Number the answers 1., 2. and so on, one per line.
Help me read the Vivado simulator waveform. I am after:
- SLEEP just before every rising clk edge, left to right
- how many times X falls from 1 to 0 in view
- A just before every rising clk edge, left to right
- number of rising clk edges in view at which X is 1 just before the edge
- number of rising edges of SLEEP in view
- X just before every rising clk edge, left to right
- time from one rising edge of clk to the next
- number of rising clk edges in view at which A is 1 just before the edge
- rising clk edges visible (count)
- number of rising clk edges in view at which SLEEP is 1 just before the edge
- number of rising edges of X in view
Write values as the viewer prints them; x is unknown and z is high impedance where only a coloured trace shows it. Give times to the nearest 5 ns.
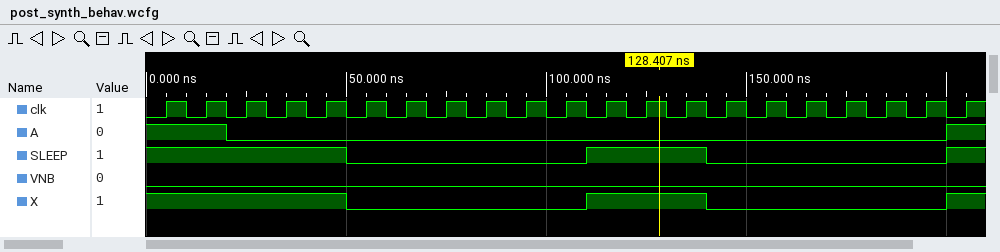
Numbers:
1. 1 1 1 1 1 0 0 0 0 0 0 1 1 1 0 0 0 0 0 0 1
2. 2
3. 1 1 0 0 0 0 0 0 0 0 0 0 0 0 0 0 0 0 0 0 1
4. 9
5. 2
6. 1 1 1 1 1 0 0 0 0 0 0 1 1 1 0 0 0 0 0 0 1
7. 10 ns
8. 3
9. 21
10. 9
11. 2
